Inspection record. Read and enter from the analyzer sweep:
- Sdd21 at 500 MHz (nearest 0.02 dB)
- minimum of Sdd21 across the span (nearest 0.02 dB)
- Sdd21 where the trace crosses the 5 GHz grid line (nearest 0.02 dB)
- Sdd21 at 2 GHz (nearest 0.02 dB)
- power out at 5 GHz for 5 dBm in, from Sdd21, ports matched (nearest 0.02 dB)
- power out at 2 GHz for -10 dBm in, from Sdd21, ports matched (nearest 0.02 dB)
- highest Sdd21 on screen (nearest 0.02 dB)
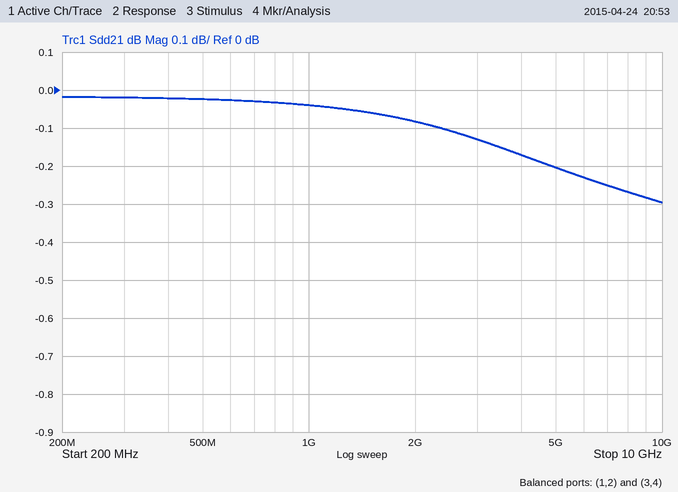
-0.02 dB
-0.30 dB
-0.20 dB
-0.08 dB
4.80 dBm
-10.08 dBm
-0.02 dB
